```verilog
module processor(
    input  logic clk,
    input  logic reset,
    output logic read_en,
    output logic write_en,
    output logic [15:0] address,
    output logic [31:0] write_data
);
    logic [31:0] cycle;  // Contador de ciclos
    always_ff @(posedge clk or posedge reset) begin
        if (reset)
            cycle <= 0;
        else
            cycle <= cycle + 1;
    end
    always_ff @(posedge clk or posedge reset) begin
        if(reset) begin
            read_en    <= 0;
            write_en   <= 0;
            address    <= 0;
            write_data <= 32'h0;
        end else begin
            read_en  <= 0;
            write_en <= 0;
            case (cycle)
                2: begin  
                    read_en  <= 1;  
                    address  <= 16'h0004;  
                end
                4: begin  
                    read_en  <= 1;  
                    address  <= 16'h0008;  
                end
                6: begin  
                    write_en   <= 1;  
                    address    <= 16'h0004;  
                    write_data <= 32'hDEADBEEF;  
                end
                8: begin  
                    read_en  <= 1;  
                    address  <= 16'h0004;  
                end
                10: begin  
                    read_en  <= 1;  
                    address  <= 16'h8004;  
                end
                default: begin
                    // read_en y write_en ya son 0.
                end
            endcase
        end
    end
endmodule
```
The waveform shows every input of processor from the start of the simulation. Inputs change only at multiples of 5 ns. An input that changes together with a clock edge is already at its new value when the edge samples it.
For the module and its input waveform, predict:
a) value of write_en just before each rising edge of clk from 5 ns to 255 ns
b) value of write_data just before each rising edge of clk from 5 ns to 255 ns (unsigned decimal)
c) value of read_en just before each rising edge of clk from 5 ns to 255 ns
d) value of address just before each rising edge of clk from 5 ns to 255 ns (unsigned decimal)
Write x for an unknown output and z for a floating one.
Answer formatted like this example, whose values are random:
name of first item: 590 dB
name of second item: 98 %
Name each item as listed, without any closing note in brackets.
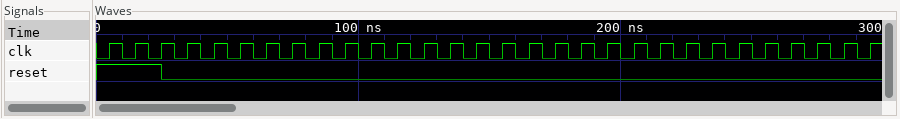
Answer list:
value of write_en just before each rising edge of clk from 5 ns to 255 ns: 0 0 0 0 0 0 0 0 0 1 0 0 0 0 0 0 0 0 0 0 0 0 0 0 0 0
value of write_data just before each rising edge of clk from 5 ns to 255 ns: 0, 0, 0, 0, 0, 0, 0, 0, 0, 3735928559, 3735928559, 3735928559, 3735928559, 3735928559, 3735928559, 3735928559, 3735928559, 3735928559, 3735928559, 3735928559, 3735928559, 3735928559, 3735928559, 3735928559, 3735928559, 3735928559
value of read_en just before each rising edge of clk from 5 ns to 255 ns: 0 0 0 0 0 1 0 1 0 0 0 1 0 1 0 0 0 0 0 0 0 0 0 0 0 0
value of address just before each rising edge of clk from 5 ns to 255 ns: 0, 0, 0, 0, 0, 4, 4, 8, 8, 4, 4, 4, 4, 32772, 32772, 32772, 32772, 32772, 32772, 32772, 32772, 32772, 32772, 32772, 32772, 32772
